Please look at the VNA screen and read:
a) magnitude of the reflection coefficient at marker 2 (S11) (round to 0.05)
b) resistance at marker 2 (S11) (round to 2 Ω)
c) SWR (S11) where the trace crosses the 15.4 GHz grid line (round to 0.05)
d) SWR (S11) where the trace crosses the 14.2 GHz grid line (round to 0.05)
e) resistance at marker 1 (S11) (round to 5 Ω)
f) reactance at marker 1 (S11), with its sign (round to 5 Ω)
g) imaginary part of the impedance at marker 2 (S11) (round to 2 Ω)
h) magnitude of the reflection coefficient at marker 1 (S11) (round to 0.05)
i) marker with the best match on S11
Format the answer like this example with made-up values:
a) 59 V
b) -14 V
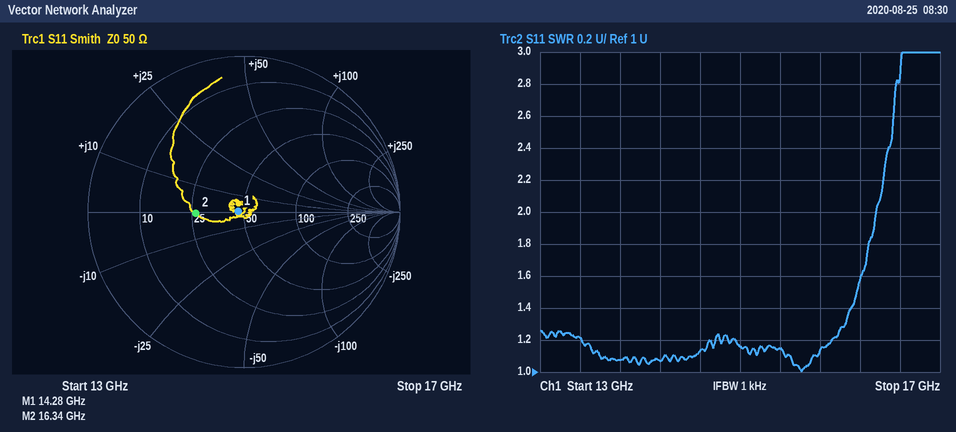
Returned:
a) 0.30
b) 26 Ω
c) 1.15
d) 1.05
e) 45 Ω
f) 0 Ω
g) 0 Ω
h) 0.05
i) marker 1
